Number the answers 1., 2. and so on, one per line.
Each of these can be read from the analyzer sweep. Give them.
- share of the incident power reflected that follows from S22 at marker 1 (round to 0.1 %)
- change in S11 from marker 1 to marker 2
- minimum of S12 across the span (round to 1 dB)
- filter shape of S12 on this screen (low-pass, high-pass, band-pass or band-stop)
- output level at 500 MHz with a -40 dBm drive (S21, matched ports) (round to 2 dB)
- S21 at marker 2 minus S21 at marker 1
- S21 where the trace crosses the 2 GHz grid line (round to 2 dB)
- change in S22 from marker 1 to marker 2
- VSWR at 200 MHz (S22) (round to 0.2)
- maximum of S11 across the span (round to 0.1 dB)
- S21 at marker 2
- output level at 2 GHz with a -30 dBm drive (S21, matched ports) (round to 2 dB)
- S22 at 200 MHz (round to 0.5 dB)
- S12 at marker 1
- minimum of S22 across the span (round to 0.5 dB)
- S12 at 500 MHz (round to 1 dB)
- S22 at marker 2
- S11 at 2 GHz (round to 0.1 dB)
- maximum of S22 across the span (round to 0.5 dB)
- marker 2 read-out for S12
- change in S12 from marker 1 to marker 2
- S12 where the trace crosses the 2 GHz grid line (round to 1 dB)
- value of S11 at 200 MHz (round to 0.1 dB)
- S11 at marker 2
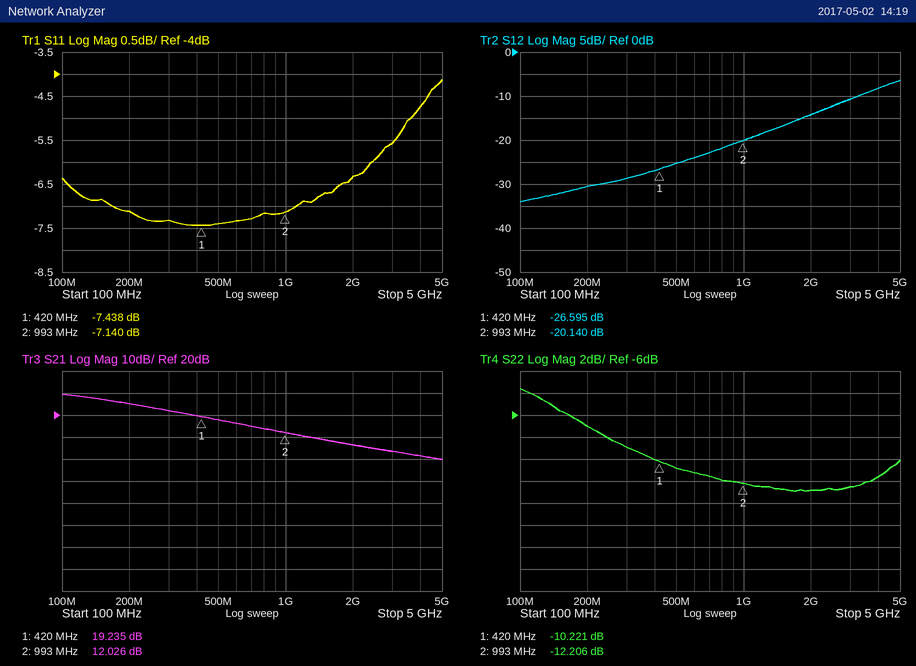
1. 9.5 %
2. 0.298 dB
3. -34 dB
4. high-pass
5. -22 dBm
6. -7.209 dB
7. 6 dB
8. -1.985 dB
9. 2.6
10. -4.1 dB
11. 12.026 dB
12. -24 dBm
13. -7.0 dB
14. -26.595 dB
15. -13.0 dB
16. -25 dB
17. -12.206 dB
18. -6.3 dB
19. -3.5 dB
20. -20.140 dB
21. 6.455 dB
22. -14 dB
23. -7.1 dB
24. -7.140 dB
